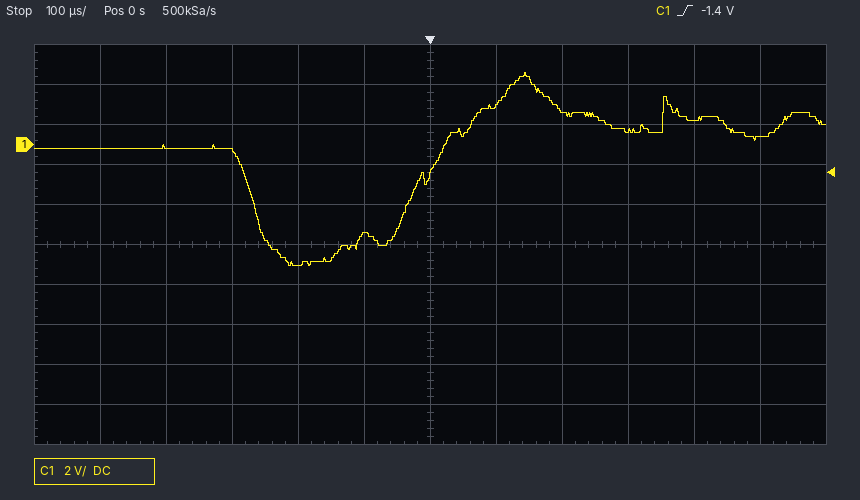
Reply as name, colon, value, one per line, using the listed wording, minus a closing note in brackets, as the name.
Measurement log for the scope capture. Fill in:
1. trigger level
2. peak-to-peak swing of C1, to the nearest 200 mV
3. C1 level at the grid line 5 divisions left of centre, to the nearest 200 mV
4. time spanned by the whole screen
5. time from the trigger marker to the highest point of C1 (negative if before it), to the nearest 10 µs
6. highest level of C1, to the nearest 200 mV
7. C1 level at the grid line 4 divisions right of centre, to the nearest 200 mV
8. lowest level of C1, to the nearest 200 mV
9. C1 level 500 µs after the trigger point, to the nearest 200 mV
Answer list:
trigger level: -1.4 V
peak-to-peak swing of C1, to the nearest 200 mV: 9.6 V
C1 level at the grid line 5 divisions left of centre, to the nearest 200 mV: -200 mV
time spanned by the whole screen: 1.2 ms
time from the trigger marker to the highest point of C1 (negative if before it), to the nearest 10 µs: +140 µs
highest level of C1, to the nearest 200 mV: 3.6 V
C1 level at the grid line 4 divisions right of centre, to the nearest 200 mV: 1.2 V
lowest level of C1, to the nearest 200 mV: -6.0 V
C1 level 500 µs after the trigger point, to the nearest 200 mV: 400 mV
